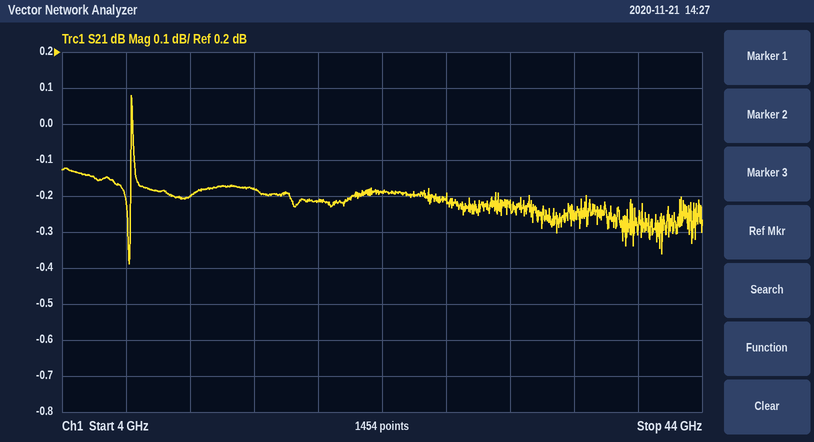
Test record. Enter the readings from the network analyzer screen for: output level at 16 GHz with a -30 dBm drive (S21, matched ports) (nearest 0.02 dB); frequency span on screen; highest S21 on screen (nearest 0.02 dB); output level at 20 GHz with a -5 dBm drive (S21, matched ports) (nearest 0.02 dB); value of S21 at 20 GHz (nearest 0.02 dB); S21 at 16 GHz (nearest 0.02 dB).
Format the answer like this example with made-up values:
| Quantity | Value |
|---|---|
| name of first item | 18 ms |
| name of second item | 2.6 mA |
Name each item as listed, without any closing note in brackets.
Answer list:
| Quantity | Value |
|---|---|
| output level at 16 GHz with a -30 dBm drive (S21, matched ports) | -30.18 dBm |
| frequency span on screen | 40 GHz |
| highest S21 on screen | 0.08 dB |
| output level at 20 GHz with a -5 dBm drive (S21, matched ports) | -5.22 dBm |
| value of S21 at 20 GHz | -0.22 dB |
| S21 at 16 GHz | -0.18 dB |
